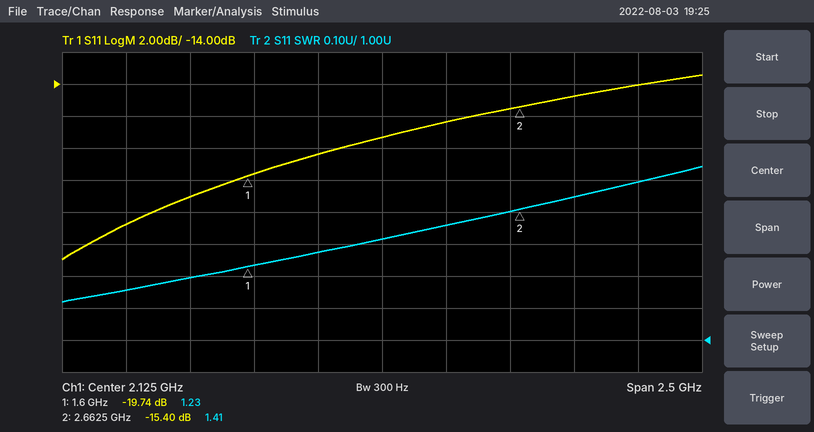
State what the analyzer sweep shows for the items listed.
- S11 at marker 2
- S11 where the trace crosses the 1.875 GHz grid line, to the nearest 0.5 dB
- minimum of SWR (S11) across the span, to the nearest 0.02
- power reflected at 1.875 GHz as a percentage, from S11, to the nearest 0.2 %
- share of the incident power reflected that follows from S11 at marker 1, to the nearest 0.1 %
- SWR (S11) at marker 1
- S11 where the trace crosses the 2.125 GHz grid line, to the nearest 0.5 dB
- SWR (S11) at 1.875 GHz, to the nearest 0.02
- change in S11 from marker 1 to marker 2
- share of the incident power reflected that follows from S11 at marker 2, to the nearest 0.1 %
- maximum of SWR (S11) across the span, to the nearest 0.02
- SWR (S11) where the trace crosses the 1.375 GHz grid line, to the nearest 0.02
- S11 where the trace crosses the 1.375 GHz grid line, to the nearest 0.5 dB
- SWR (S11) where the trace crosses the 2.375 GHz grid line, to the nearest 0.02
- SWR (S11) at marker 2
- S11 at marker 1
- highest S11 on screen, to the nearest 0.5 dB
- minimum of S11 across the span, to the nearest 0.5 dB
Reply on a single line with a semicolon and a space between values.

-15.40 dB; -18.5 dB; 1.12; 1.4 %; 1.1 %; 1.23; -17.5 dB; 1.28; 4.34 dB; 2.9 %; 1.54; 1.20; -21.0 dB; 1.36; 1.41; -19.74 dB; -13.5 dB; -25.0 dB
